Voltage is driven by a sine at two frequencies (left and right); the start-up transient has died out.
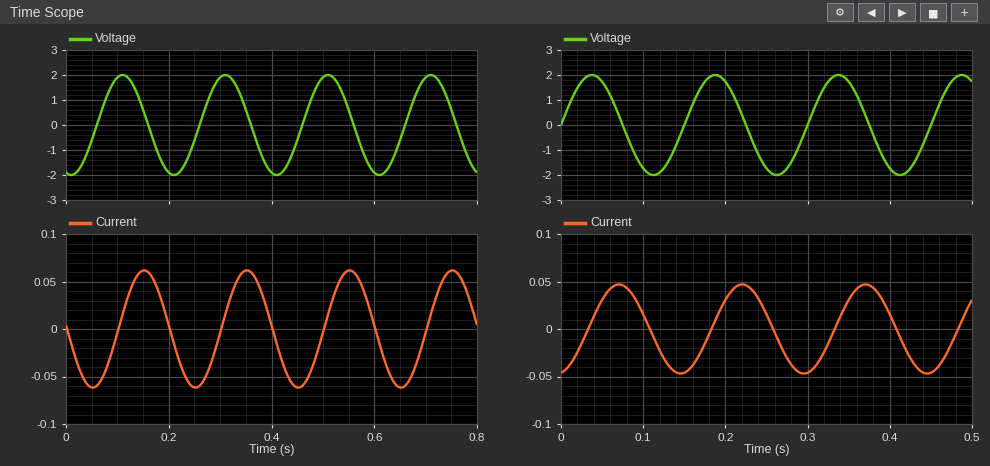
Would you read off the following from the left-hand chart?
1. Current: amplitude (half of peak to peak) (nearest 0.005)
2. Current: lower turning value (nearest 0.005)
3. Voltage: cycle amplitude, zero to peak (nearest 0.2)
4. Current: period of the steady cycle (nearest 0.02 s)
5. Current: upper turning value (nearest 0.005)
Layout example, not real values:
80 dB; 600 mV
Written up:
0.060; -0.060; 2.0; 0.20 s; 0.060
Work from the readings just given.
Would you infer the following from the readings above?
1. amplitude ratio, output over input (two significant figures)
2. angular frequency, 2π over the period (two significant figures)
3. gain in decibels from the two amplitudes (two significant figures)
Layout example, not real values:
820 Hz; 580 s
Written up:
0.030; 31 rad/s; -30 dB
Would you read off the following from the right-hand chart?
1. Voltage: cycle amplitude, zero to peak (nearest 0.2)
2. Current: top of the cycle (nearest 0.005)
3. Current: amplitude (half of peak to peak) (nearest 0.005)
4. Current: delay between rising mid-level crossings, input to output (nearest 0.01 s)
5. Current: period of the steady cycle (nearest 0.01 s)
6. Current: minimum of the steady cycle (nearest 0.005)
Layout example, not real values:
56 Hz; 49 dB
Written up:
2.0; 0.045; 0.045; 0.03 s; 0.15 s; -0.045
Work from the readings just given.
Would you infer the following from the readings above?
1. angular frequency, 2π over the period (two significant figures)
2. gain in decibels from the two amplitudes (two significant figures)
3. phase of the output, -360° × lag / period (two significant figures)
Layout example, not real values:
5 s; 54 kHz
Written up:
42 rad/s; -33 dB; -72°
